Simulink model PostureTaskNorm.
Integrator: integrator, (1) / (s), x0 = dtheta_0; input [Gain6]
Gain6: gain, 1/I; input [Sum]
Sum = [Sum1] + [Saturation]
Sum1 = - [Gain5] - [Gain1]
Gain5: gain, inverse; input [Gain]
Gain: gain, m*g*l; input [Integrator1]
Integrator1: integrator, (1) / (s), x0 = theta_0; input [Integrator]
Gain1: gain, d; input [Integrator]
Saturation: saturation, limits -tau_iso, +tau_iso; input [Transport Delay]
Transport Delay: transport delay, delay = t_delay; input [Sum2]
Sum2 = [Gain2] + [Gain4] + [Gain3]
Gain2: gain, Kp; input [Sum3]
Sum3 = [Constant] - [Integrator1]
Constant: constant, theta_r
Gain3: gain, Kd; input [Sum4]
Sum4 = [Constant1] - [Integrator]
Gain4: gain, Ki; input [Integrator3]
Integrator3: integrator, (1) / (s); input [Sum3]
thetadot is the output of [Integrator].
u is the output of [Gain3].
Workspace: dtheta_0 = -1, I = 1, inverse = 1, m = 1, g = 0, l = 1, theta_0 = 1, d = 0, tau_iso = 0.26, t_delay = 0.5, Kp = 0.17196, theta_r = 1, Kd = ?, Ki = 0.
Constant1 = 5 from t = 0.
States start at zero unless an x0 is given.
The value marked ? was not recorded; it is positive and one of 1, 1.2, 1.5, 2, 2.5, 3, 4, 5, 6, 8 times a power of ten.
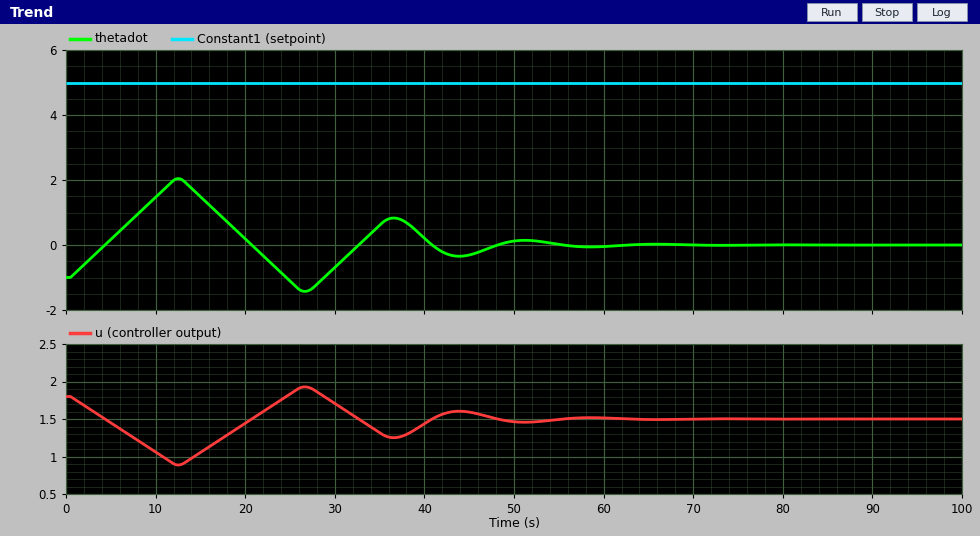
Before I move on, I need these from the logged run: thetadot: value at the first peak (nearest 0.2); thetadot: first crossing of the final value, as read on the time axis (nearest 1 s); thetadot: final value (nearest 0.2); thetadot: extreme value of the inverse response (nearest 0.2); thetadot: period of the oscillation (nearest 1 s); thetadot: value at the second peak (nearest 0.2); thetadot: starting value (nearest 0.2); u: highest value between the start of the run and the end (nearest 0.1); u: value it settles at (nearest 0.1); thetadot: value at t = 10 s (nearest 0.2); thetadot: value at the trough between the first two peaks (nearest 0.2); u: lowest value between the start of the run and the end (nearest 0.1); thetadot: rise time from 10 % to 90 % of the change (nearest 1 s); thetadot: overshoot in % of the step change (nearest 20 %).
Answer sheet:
2.0
4 s
0.0
-1.4
24 s
0.8
-1.0
1.9
1.5
1.4
-1.4
0.9
3 s
200 %
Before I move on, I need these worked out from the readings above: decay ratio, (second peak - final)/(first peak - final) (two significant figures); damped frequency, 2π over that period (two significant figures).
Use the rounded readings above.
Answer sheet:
0.40
0.26 rad/s
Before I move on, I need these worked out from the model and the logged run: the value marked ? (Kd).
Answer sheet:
0.3
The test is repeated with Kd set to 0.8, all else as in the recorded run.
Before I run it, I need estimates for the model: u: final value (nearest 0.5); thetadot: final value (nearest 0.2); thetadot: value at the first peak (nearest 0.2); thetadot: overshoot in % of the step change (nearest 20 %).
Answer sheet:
4.0
0.0
2.8
280 %
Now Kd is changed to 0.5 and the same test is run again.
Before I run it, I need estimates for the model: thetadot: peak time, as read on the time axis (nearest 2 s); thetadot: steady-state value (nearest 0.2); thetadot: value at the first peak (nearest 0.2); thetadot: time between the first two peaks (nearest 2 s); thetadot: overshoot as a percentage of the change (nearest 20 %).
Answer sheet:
14 s
0.0
2.4
22 s
240 %
